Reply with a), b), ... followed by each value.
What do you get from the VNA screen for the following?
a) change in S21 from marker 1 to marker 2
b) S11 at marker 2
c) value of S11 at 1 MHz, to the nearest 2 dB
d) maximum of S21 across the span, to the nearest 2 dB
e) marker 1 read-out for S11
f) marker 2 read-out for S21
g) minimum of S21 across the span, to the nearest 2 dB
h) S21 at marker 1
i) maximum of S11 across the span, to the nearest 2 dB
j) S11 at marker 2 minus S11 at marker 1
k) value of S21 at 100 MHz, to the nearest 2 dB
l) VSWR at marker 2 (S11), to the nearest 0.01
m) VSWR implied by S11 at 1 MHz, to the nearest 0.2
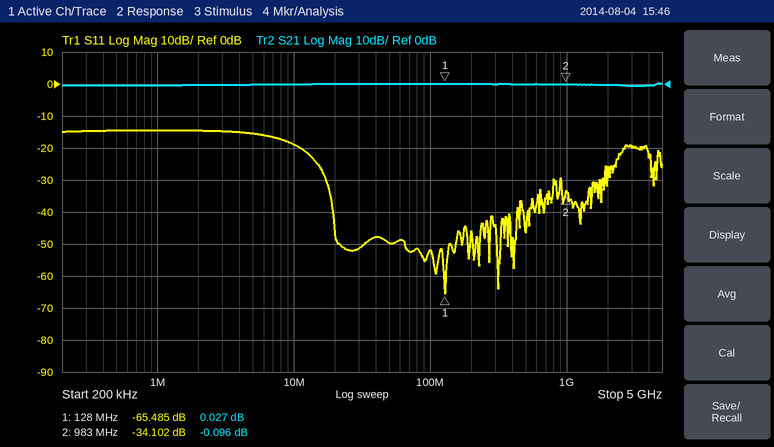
a) -0.123 dB
b) -34.102 dB
c) -14 dB
d) 0 dB
e) -65.485 dB
f) -0.096 dB
g) 0 dB
h) 0.027 dB
i) -14 dB
j) 31.383 dB
k) 0 dB
l) 1.04
m) 1.4
